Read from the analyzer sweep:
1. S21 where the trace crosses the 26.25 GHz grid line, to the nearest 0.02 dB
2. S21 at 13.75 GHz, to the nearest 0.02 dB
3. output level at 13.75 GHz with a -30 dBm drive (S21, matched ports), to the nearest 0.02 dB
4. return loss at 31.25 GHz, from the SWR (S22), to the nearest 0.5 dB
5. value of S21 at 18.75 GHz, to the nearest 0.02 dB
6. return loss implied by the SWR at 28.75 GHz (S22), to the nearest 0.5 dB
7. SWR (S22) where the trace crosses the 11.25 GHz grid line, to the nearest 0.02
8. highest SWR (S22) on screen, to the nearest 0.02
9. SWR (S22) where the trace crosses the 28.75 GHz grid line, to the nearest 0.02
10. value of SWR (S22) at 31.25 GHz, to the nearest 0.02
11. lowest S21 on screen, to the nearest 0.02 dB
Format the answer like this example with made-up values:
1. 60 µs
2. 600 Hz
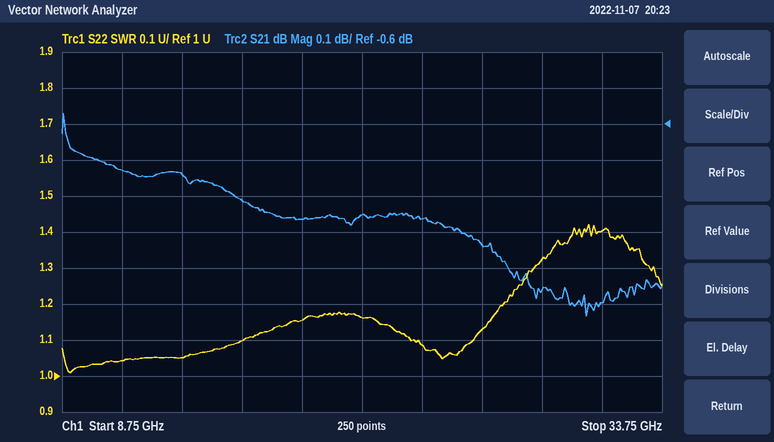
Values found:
1. -0.94 dB
2. -0.74 dB
3. -30.74 dBm
4. 15.5 dB
5. -0.86 dB
6. 17.0 dB
7. 1.04
8. 1.42
9. 1.32
10. 1.40
11. -1.14 dB
